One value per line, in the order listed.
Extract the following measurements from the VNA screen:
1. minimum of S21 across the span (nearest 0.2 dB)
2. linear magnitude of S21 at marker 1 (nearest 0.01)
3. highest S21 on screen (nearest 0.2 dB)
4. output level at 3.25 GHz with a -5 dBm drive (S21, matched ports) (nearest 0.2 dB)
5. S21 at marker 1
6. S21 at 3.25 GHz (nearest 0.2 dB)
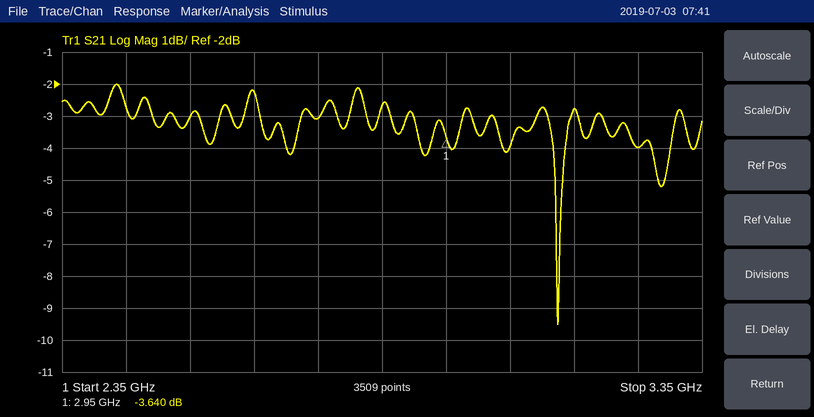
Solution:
-9.6 dB
0.66
-2.0 dB
-9.0 dBm
-3.640 dB
-4.0 dB
